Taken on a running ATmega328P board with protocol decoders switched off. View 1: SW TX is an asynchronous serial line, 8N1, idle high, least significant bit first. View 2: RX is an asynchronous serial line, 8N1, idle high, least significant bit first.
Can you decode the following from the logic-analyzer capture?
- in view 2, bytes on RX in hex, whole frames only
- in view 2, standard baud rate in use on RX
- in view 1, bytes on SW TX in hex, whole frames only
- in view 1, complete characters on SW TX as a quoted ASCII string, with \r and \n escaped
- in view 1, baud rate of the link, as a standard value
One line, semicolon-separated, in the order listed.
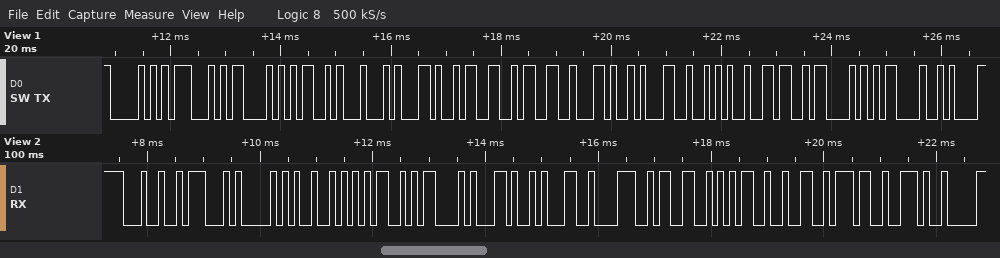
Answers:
24 47 50 52 4D 43 2C 31 38 33 35 32 37 2E; 9600 baud; 50 47 43 4D 44 2C 33 33 2C 31 2A 36 43 0D 0A; "PGCMD,33,1*6C\r\n"; 9600 baud
